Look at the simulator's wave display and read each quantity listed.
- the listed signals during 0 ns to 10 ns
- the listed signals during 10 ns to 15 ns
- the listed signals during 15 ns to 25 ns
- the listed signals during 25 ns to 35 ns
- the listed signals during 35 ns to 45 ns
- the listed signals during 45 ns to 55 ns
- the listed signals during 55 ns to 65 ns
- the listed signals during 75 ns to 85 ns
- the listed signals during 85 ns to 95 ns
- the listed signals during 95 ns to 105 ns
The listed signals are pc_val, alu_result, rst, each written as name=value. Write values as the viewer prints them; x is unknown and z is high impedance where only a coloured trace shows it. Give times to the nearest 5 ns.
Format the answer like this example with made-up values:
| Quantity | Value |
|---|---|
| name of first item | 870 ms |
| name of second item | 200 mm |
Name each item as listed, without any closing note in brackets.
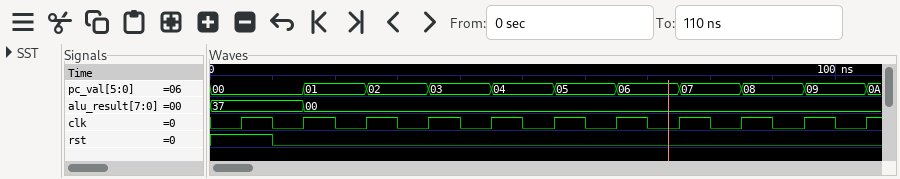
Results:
| Quantity | Value |
|---|---|
| the listed signals during 0 ns to 10 ns | pc_val=00, alu_result=37, rst=1 |
| the listed signals during 10 ns to 15 ns | pc_val=00, alu_result=37, rst=0 |
| the listed signals during 15 ns to 25 ns | pc_val=01, alu_result=00, rst=0 |
| the listed signals during 25 ns to 35 ns | pc_val=02, alu_result=00, rst=0 |
| the listed signals during 35 ns to 45 ns | pc_val=03, alu_result=00, rst=0 |
| the listed signals during 45 ns to 55 ns | pc_val=04, alu_result=00, rst=0 |
| the listed signals during 55 ns to 65 ns | pc_val=05, alu_result=00, rst=0 |
| the listed signals during 75 ns to 85 ns | pc_val=07, alu_result=00, rst=0 |
| the listed signals during 85 ns to 95 ns | pc_val=08, alu_result=00, rst=0 |
| the listed signals during 95 ns to 105 ns | pc_val=09, alu_result=00, rst=0 |
